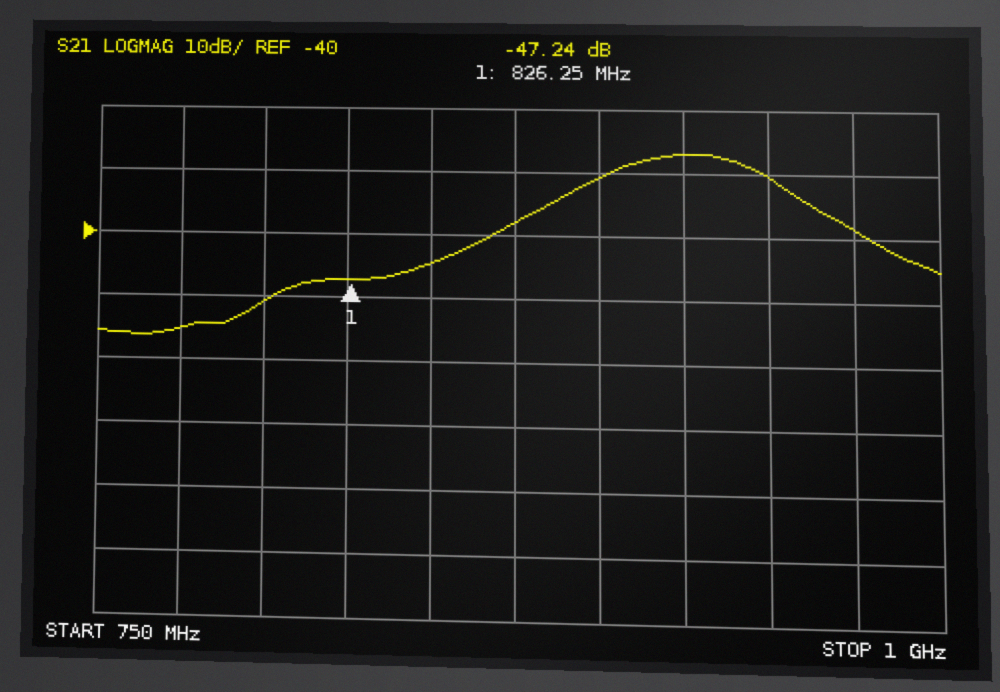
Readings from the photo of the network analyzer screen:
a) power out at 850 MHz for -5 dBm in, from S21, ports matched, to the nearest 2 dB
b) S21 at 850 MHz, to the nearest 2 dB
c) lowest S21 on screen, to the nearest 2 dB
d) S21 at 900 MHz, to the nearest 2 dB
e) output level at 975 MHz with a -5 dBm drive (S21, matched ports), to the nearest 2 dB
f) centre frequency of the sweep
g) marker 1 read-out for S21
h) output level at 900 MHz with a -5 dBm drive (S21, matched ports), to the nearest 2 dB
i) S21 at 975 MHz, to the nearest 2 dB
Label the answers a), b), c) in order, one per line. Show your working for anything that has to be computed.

a) -5 dBm + (-44 dB) = -50 dBm
b) -44 dB
c) -56 dB
d) -30 dB
e) -5 dBm + (-38 dB) = -44 dBm
f) 875 MHz
g) -47.24 dB
h) -5 dBm + (-30 dB) = -36 dBm
i) -38 dB
